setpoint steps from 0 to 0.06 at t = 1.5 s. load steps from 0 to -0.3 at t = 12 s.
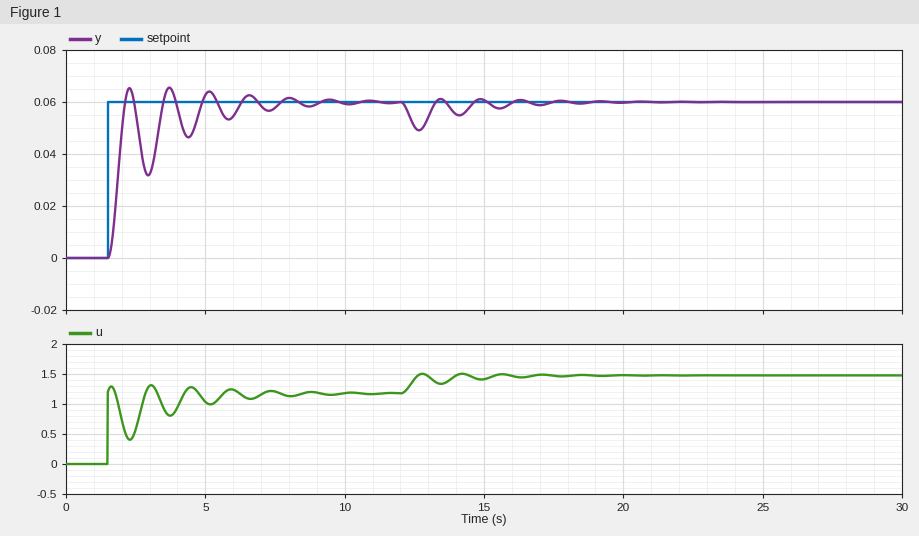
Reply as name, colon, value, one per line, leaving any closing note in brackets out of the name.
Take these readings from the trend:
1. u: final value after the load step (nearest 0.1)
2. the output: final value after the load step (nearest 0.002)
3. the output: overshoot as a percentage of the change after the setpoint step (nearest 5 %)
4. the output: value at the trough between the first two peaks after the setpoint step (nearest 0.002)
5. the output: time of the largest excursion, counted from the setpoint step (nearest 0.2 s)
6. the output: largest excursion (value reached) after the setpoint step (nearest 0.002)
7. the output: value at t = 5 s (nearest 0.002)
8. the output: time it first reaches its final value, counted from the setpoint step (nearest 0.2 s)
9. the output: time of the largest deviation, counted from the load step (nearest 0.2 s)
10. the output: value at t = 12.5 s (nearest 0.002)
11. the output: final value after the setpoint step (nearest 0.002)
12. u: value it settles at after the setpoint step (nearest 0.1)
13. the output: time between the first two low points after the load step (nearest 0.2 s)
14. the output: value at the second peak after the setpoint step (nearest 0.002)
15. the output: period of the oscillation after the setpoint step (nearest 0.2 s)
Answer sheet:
u: final value after the load step: 1.5
the output: final value after the load step: 0.060
the output: overshoot as a percentage of the change after the setpoint step: 10 %
the output: value at the trough between the first two peaks after the setpoint step: 0.032
the output: time of the largest excursion, counted from the setpoint step: 2.2 s
the output: largest excursion (value reached) after the setpoint step: 0.066
the output: value at t = 5 s: 0.062
the output: time it first reaches its final value, counted from the setpoint step: 0.6 s
the output: time of the largest deviation, counted from the load step: 0.6 s
the output: value at t = 12.5 s: 0.050
the output: final value after the setpoint step: 0.060
u: value it settles at after the setpoint step: 1.2
the output: time between the first two low points after the load step: 1.4 s
the output: value at the second peak after the setpoint step: 0.066
the output: period of the oscillation after the setpoint step: 1.4 s
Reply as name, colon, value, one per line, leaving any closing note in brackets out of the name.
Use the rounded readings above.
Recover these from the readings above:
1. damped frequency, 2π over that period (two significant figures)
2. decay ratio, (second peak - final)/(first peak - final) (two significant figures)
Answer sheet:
damped frequency, 2π over that period: 4.5 rad/s
decay ratio, (second peak - final)/(first peak - final): 1.0
